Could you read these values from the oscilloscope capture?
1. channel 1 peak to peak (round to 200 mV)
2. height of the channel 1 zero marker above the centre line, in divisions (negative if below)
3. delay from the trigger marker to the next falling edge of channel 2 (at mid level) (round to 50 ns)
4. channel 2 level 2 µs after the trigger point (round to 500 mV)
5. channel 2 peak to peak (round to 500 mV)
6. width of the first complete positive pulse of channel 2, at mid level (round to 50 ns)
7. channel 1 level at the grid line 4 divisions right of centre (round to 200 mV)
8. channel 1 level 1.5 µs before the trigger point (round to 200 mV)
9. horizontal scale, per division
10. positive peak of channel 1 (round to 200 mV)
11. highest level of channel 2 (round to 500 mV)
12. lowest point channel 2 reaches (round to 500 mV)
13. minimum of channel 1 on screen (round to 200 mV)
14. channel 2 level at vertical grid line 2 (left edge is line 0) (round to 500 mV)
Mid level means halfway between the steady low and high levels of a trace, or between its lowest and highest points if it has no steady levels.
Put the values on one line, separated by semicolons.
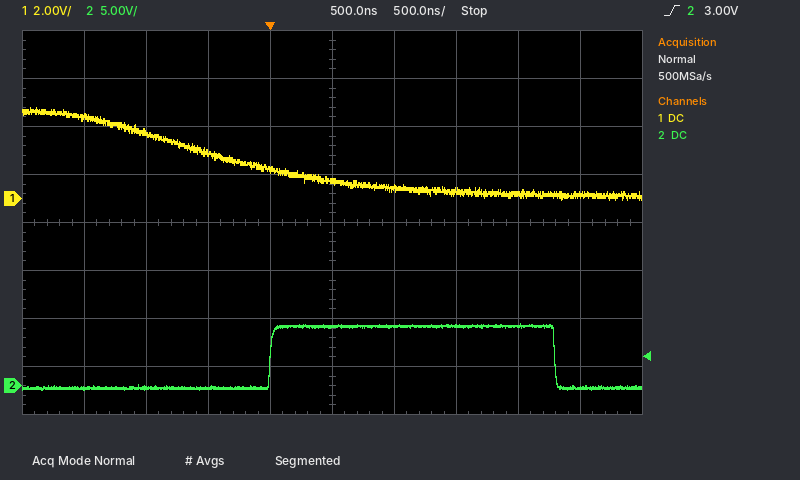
3.8 V; +0.5 div; 2.30 µs; 6.5 V; 7.0 V; 2.30 µs; 200 mV; 3.4 V; 500 ns; 3.8 V; 6.5 V; -500 mV; 0.0 V; 0.0 V
